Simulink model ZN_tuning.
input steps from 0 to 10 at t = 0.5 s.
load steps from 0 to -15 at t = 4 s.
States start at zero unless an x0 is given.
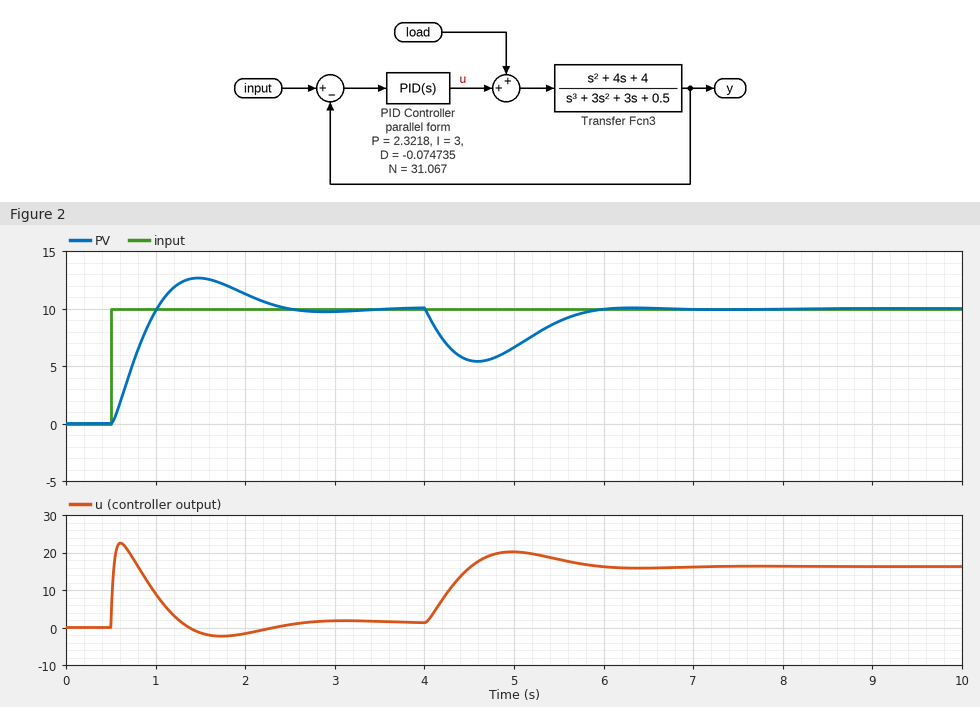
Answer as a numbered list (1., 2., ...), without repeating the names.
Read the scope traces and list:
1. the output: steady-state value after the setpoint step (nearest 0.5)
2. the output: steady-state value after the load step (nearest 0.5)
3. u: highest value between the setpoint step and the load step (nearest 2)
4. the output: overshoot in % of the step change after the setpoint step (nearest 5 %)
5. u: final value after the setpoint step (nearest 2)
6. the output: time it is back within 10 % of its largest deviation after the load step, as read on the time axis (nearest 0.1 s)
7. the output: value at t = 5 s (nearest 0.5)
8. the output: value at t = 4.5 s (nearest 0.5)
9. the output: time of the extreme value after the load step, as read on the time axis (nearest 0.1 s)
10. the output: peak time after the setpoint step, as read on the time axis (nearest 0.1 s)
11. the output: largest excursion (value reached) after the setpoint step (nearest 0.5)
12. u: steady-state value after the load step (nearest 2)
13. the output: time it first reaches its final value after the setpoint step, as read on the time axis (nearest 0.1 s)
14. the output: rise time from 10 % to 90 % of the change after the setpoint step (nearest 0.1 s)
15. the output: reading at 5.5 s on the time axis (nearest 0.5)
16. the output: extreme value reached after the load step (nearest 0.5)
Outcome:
1. 10.0
2. 10.0
3. 22
4. 25 %
5. 2
6. 5.7 s
7. 6.5
8. 5.5
9. 4.6 s
10. 1.5 s
11. 12.5
12. 16
13. 1.0 s
14. 0.4 s
15. 9.0
16. 5.5
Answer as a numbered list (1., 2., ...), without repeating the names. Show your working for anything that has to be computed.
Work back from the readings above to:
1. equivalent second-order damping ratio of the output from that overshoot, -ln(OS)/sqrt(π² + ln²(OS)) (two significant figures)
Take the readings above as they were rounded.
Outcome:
1. ln(0.25) = -1.386; 1.386 / sqrt(9.870 + 1.922) = 0.40
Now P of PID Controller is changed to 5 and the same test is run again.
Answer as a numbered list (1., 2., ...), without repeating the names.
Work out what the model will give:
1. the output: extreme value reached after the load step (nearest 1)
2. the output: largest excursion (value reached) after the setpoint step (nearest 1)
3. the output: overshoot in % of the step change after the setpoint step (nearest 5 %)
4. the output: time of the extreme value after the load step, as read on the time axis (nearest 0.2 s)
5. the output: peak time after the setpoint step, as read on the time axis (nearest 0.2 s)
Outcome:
1. 7
2. 11
3. 10 %
4. 4.4 s
5. 1.2 s
